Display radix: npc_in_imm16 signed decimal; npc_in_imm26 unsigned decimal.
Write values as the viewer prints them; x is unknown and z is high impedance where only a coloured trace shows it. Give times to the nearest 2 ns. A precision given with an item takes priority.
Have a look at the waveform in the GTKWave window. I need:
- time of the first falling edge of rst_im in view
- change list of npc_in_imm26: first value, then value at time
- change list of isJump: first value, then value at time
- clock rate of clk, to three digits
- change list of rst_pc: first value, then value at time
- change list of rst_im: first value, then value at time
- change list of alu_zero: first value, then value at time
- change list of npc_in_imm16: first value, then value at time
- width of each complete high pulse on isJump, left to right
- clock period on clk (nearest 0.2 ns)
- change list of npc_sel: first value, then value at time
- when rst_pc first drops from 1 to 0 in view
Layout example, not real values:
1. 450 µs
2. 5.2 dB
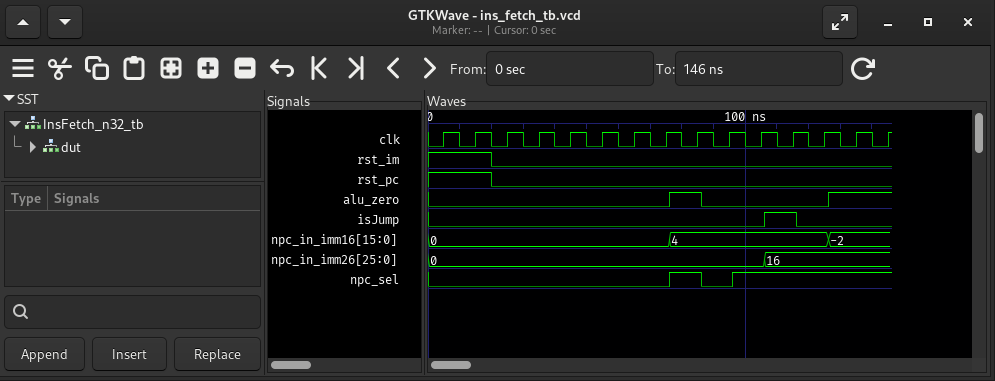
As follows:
1. 20 ns
2. 0, 16 at 106 ns
3. 0, 1 at 106 ns, 0 at 116 ns
4. 100 MHz
5. 1, 0 at 20 ns
6. 1, 0 at 20 ns
7. 0, 1 at 76 ns, 0 at 86 ns, 1 at 126 ns
8. 0, 4 at 76 ns, -2 at 126 ns
9. 10 ns
10. 10 ns
11. 0, 1 at 76 ns, 0 at 86 ns, 1 at 96 ns
12. 20 ns
